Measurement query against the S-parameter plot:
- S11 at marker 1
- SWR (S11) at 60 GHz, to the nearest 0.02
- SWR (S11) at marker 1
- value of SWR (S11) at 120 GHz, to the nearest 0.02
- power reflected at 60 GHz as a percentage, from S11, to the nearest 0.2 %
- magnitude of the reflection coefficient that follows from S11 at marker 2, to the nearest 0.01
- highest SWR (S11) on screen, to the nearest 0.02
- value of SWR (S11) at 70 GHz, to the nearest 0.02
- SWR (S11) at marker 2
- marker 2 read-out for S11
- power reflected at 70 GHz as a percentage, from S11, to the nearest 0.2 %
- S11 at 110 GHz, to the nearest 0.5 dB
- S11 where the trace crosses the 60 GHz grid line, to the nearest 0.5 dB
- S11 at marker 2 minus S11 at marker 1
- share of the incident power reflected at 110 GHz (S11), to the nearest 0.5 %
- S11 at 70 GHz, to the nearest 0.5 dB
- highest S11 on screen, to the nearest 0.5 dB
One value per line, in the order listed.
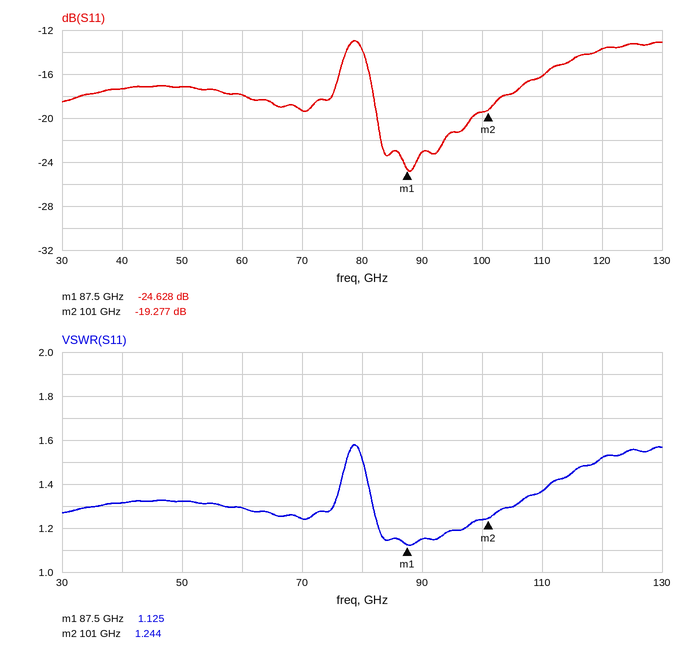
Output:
-24.628 dB
1.30
1.125
1.52
1.6 %
0.11
1.58
1.24
1.244
-19.277 dB
1.2 %
-16.0 dB
-18.0 dB
5.351 dB
2.5 %
-19.5 dB
-13.0 dB
